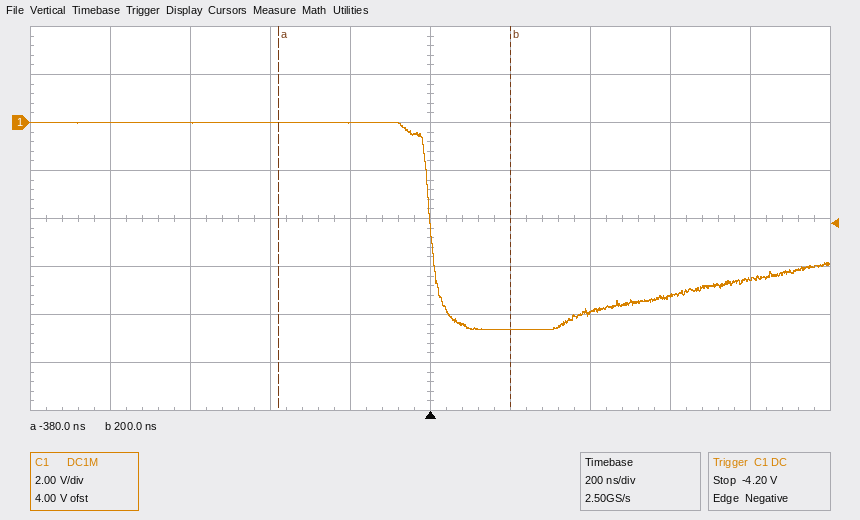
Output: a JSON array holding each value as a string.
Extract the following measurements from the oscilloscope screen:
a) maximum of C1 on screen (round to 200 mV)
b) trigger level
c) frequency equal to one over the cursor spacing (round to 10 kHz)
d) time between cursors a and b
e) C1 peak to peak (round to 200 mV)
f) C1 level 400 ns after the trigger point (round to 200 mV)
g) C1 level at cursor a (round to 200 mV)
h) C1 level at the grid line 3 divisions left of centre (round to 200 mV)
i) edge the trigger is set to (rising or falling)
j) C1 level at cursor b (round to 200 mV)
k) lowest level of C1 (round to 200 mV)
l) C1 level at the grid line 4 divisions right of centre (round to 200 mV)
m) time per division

["0.0 V", "-4.20 V", "1.72 MHz", "580 ns", "8.6 V", "-8.0 V", "0.0 V", "0.0 V", "falling", "-8.6 V", "-8.6 V", "-6.6 V", "200 ns"]
